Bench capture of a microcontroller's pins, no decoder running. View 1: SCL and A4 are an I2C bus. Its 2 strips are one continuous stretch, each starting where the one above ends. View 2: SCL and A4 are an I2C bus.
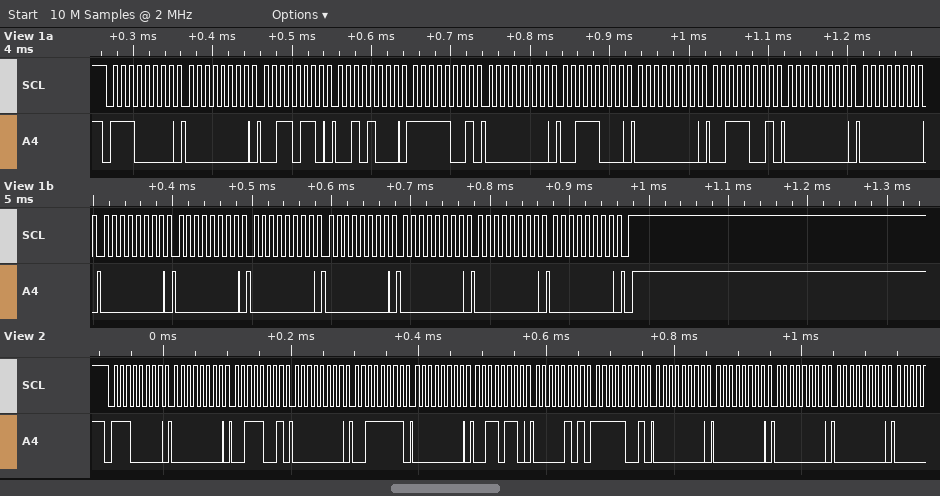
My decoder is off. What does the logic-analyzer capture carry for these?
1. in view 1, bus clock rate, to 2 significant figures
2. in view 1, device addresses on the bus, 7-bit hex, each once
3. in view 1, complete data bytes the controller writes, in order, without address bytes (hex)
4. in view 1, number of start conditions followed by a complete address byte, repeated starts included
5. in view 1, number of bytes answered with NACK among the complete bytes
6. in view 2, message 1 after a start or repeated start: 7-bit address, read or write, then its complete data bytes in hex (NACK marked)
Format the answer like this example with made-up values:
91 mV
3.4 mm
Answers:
100 kHz
0x70
00 36 28 F9 00 38 00 39 00 00 00 00 00 00 00 00 00
1
0
0x70 write: 00 39 00 3F 00 36 05 F9 00 00 00 00
